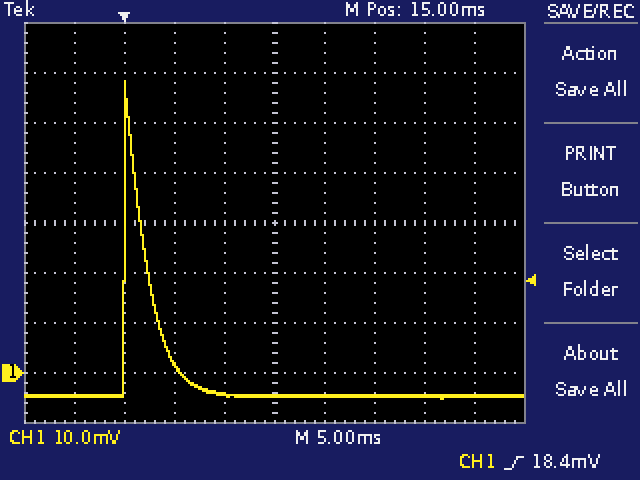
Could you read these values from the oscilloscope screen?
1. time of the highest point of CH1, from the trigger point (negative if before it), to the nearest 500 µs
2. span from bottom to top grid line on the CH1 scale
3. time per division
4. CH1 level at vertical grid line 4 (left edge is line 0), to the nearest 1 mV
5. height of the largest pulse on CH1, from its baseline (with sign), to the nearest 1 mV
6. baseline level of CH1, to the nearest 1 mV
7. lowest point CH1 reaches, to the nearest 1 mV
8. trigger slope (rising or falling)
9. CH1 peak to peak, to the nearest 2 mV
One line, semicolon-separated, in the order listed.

0.0 ms; 80 mV; 5 ms; -4 mV; +63 mV; -5 mV; -5 mV; rising; 64 mV
